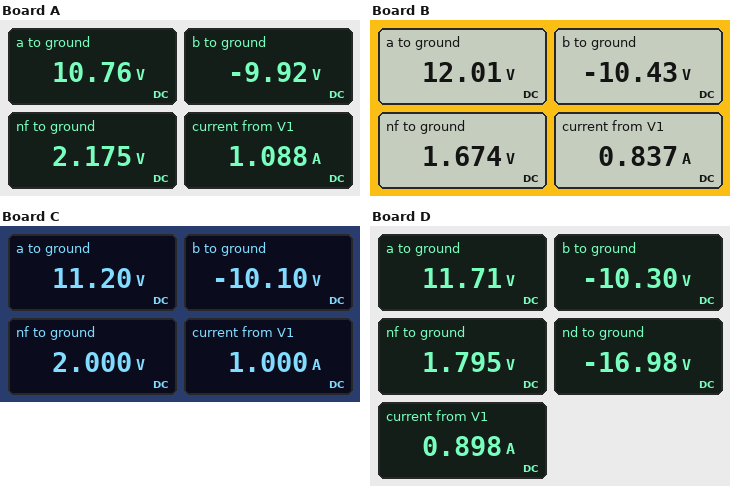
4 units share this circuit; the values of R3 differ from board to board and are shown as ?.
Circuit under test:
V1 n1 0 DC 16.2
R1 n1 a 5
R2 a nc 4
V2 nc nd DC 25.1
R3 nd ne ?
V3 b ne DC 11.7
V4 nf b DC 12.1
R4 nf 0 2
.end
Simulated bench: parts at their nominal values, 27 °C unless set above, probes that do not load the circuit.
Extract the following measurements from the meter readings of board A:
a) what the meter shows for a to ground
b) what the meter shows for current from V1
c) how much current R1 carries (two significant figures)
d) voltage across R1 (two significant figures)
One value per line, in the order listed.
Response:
10.76 V
1.088 A
1.1 A
5.4 V
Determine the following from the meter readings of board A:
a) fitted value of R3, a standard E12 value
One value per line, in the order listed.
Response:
2.7 Ω
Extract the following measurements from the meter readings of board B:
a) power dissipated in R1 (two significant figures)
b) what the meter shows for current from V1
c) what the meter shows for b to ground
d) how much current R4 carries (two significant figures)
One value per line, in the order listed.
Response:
3.5 W
0.837 A
-10.43 V
840 mA
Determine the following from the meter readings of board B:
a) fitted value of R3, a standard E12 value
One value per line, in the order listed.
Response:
6.8 Ω
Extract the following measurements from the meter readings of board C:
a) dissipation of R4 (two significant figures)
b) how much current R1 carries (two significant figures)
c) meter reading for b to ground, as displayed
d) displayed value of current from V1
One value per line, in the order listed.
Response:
2.0 W
1.0 A
-10.10 V
1.000 A
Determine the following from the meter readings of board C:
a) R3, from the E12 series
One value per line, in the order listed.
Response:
3.9 Ω
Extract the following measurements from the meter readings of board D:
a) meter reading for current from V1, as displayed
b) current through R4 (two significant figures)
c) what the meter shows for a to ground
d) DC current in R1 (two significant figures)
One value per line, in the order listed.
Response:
0.898 A
900 mA
11.71 V
900 mA
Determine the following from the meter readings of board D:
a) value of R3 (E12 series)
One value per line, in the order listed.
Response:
5.6 Ω
